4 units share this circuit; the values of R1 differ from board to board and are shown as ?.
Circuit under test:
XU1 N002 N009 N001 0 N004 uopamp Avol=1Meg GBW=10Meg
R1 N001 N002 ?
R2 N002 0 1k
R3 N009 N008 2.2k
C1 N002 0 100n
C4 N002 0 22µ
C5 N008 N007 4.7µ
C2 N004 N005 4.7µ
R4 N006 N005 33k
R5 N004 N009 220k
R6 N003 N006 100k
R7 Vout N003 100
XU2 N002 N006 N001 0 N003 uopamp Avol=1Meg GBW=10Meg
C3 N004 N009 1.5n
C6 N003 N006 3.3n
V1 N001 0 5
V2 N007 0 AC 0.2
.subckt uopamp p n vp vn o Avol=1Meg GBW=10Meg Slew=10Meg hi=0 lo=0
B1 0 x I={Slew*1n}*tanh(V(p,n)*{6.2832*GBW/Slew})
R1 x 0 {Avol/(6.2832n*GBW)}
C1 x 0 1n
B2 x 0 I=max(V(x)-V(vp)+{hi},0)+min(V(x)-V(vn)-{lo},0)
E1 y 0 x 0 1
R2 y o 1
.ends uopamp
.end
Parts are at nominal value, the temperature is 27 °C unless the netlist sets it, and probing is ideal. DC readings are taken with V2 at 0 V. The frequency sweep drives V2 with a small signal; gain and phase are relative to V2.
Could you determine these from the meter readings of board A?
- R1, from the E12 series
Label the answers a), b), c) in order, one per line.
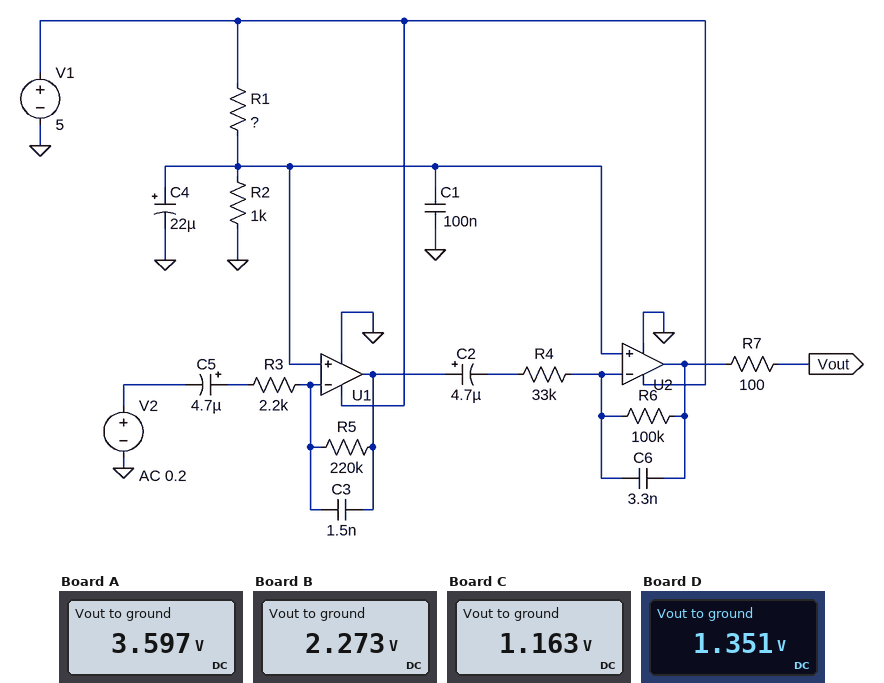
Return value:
a) 390 Ω
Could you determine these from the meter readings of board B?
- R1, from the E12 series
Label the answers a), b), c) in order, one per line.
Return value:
a) 1.2 kΩ
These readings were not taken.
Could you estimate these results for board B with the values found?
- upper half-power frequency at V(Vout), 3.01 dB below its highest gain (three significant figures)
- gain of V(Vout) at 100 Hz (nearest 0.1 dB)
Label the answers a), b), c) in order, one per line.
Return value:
a) 332 Hz
b) 49.2 dB
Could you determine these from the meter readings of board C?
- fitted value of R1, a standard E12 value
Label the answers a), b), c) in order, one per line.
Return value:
a) 3.3 kΩ
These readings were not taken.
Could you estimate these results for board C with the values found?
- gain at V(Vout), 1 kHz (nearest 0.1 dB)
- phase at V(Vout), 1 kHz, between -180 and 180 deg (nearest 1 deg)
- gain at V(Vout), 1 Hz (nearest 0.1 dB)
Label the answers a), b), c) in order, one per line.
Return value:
a) 35.1 dB
b) -128 deg
c) 22.7 dB
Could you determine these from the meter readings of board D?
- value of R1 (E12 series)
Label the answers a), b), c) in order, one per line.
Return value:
a) 2.7 kΩ
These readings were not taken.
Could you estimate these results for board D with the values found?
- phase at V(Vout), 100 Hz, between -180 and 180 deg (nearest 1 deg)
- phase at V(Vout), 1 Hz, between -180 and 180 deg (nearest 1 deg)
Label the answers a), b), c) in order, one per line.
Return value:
a) -14 deg
b) 132 deg
